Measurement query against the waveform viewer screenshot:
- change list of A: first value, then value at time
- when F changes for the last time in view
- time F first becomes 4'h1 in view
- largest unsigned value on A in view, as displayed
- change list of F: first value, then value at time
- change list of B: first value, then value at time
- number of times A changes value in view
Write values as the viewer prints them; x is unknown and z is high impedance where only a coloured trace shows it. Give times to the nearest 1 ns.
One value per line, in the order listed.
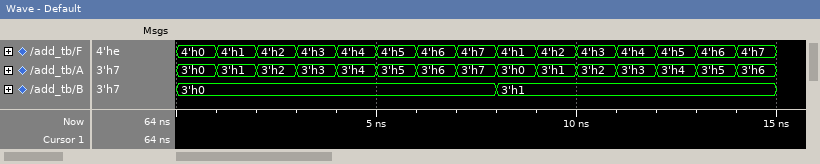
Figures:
3'h0, 3'h1 at 1 ns, 3'h2 at 2 ns, 3'h3 at 3 ns, 3'h4 at 4 ns, 3'h5 at 5 ns, 3'h6 at 6 ns, 3'h7 at 7 ns, 3'h0 at 8 ns, 3'h1 at 9 ns, 3'h2 at 10 ns, 3'h3 at 11 ns, 3'h4 at 12 ns, 3'h5 at 13 ns, 3'h6 at 14 ns
14 ns
1 ns
3'h7
4'h0, 4'h1 at 1 ns, 4'h2 at 2 ns, 4'h3 at 3 ns, 4'h4 at 4 ns, 4'h5 at 5 ns, 4'h6 at 6 ns, 4'h7 at 7 ns, 4'h1 at 8 ns, 4'h2 at 9 ns, 4'h3 at 10 ns, 4'h4 at 11 ns, 4'h5 at 12 ns, 4'h6 at 13 ns, 4'h7 at 14 ns
3'h0, 3'h1 at 8 ns
14
